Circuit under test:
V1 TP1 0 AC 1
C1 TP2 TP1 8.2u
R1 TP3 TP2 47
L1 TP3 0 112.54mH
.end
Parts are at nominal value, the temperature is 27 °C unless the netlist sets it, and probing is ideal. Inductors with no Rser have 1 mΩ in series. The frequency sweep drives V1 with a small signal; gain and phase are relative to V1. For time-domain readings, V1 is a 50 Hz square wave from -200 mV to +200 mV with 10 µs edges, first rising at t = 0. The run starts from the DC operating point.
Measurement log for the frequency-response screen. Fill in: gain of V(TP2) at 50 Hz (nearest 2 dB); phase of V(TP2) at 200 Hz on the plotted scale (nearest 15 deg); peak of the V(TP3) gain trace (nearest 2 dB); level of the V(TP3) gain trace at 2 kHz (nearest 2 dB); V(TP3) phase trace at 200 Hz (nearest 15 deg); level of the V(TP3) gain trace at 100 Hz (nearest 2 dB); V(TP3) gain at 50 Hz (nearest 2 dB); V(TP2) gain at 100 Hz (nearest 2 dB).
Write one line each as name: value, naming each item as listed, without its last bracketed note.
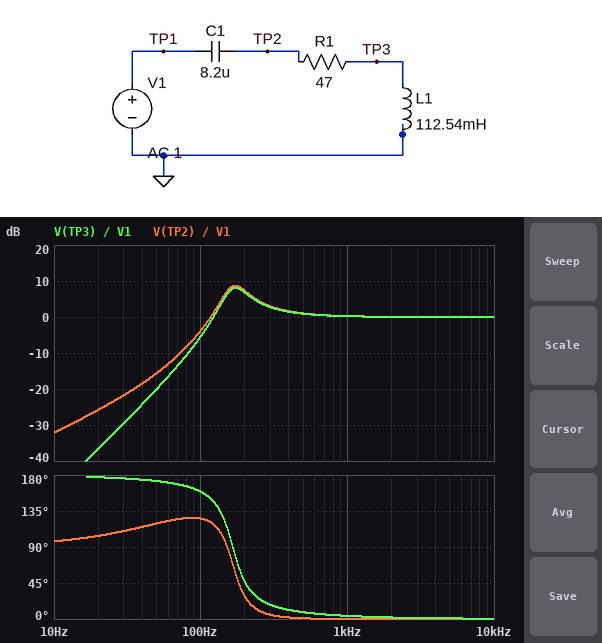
gain of V(TP2) at 50 Hz: -16 dB
phase of V(TP2) at 200 Hz on the plotted scale: 30 deg
peak of the V(TP3) gain trace: 8 dB
level of the V(TP3) gain trace at 2 kHz: 0 dB
V(TP3) phase trace at 200 Hz: 45 deg
level of the V(TP3) gain trace at 100 Hz: -6 dB
V(TP3) gain at 50 Hz: -20 dB
V(TP2) gain at 100 Hz: -4 dB
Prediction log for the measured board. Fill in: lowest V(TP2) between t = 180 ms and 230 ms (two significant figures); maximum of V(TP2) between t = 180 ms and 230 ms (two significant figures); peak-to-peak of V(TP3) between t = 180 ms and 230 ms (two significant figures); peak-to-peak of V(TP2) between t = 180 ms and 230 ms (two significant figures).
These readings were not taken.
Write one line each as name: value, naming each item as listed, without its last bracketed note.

lowest V(TP2) between t = 180 ms and 230 ms: -440 mV
maximum of V(TP2) between t = 180 ms and 230 ms: 440 mV
peak-to-peak of V(TP3) between t = 180 ms and 230 ms: 850 mV
peak-to-peak of V(TP2) between t = 180 ms and 230 ms: 890 mV
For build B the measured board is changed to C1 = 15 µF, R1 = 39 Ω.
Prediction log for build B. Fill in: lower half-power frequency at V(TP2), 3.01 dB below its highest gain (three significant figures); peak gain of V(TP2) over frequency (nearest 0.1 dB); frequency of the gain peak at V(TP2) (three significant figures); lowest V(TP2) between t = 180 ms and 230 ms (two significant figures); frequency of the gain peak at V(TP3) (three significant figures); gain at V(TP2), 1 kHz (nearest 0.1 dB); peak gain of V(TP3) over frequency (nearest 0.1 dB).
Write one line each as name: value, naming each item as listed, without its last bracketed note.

lower half-power frequency at V(TP2), 3.01 dB below its highest gain: 105 Hz
peak gain of V(TP2) over frequency: 7.9 dB
frequency of the gain peak at V(TP2): 128 Hz
lowest V(TP2) between t = 180 ms and 230 ms: -360 mV
frequency of the gain peak at V(TP3): 129 Hz
gain at V(TP2), 1 kHz: 0.1 dB
peak gain of V(TP3) over frequency: 7.2 dB
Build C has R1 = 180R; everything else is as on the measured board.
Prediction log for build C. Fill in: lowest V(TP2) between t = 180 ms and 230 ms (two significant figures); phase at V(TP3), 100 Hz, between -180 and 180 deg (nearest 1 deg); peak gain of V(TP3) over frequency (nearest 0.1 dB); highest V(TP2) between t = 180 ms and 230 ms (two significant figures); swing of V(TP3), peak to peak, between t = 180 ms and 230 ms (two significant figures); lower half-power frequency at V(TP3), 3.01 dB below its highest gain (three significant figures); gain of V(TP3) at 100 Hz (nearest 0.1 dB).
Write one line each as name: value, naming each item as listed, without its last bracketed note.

lowest V(TP2) between t = 180 ms and 230 ms: -400 mV
phase at V(TP3), 100 Hz, between -180 and 180 deg: 124 deg
peak gain of V(TP3) over frequency: 0 dB
highest V(TP2) between t = 180 ms and 230 ms: 400 mV
swing of V(TP3), peak to peak, between t = 180 ms and 230 ms: 790 mV
lower half-power frequency at V(TP3), 3.01 dB below its highest gain: 181 Hz
gain of V(TP3) at 100 Hz: -9.8 dB
